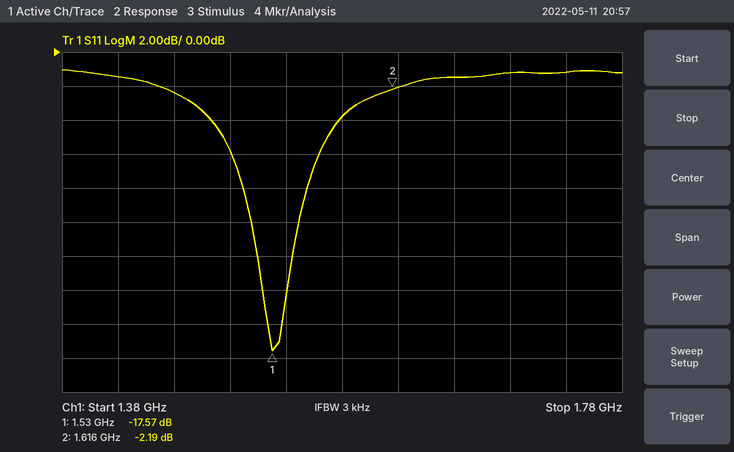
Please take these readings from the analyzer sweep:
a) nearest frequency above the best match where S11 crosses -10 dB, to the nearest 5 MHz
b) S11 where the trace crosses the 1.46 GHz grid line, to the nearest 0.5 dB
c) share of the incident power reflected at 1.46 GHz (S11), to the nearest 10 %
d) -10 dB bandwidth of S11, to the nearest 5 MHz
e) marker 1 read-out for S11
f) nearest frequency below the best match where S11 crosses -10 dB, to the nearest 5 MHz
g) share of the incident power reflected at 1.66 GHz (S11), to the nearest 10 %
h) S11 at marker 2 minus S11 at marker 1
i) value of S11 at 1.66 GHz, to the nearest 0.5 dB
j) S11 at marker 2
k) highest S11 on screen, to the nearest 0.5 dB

1.550 GHz
-2.5 dB
60 %
35 MHz
-17.57 dB
1.515 GHz
70 %
15.38 dB
-1.5 dB
-2.19 dB
-1.0 dB
